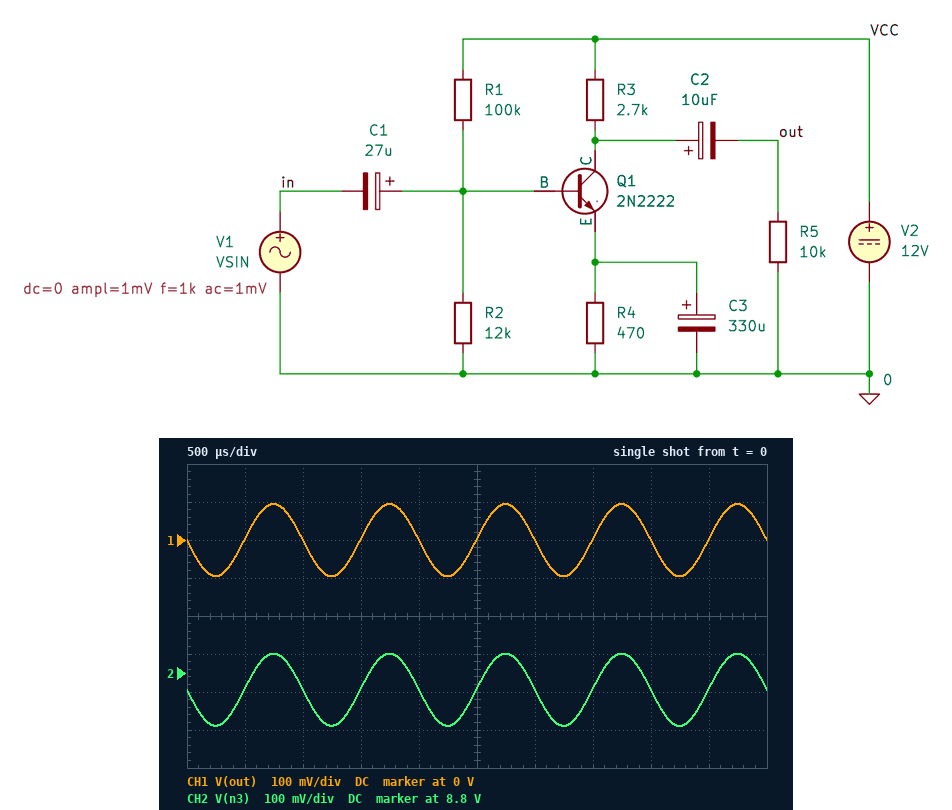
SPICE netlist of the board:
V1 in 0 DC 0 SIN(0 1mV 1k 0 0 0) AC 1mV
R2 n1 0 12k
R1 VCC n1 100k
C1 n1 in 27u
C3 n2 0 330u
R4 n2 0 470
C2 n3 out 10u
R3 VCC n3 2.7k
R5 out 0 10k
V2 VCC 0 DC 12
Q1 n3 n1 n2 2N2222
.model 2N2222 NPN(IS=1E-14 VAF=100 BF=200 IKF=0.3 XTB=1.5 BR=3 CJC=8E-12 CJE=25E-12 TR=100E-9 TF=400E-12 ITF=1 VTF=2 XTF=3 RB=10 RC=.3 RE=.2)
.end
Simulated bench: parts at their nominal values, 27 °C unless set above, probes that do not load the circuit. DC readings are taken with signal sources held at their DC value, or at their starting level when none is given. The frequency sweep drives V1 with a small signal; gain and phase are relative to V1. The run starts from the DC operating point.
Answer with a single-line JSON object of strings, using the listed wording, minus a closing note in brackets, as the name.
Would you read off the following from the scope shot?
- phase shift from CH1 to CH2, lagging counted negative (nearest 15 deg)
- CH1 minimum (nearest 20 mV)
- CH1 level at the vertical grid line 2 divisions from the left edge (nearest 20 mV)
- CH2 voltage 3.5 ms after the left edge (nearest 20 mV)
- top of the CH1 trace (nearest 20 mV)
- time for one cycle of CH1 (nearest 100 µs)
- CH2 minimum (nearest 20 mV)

{"phase shift from CH1 to CH2, lagging counted negative": "0 deg", "CH1 minimum": "-100 mV", "CH1 level at the vertical grid line 2 divisions from the left edge": "0 V", "CH2 voltage 3.5 ms after the left edge": "8.76 V", "top of the CH1 trace": "100 mV", "time for one cycle of CH1": "1.0 ms", "CH2 minimum": "8.66 V"}
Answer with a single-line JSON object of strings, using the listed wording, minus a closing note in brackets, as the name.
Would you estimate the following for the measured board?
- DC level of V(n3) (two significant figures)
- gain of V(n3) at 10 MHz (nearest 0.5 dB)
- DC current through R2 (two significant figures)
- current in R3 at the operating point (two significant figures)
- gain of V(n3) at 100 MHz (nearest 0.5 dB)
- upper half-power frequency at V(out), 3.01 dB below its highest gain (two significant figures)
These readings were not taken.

{"DC level of V(n3)": "8.8 V", "gain of V(n3) at 10 MHz": "38.0 dB", "DC current through R2": "100 µA", "current in R3 at the operating point": "1.2 mA", "gain of V(n3) at 100 MHz": "22.5 dB", "upper half-power frequency at V(out), 3.01 dB below its highest gain": "14 MHz"}
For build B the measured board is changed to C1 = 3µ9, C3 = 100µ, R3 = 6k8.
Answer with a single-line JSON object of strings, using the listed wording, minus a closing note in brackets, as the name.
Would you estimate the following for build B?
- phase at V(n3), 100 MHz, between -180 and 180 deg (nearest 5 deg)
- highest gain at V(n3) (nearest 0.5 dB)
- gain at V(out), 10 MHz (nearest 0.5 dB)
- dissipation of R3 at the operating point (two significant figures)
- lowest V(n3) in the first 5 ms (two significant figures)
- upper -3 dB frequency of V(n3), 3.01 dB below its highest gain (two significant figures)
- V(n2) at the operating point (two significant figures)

{"phase at V(n3), 100 MHz, between -180 and 180 deg": "75 deg", "highest gain at V(n3)": "45.0 dB", "gain at V(out), 10 MHz": "39.0 dB", "dissipation of R3 at the operating point": "9.7 mW", "lowest V(n3) in the first 5 ms": "3.7 V", "upper -3 dB frequency of V(n3), 3.01 dB below its highest gain": "5.8 MHz", "V(n2) at the operating point": "560 mV"}
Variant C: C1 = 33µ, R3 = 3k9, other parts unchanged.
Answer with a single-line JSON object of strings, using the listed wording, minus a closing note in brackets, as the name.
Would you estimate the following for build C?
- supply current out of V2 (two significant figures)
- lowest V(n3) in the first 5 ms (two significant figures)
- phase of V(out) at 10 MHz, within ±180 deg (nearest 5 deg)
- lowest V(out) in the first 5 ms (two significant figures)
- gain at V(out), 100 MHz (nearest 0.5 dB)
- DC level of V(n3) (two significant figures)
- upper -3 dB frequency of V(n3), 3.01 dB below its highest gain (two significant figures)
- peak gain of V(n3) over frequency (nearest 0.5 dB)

{"supply current out of V2": "1.3 mA", "lowest V(n3) in the first 5 ms": "7.2 V", "phase of V(out) at 10 MHz, within ±180 deg": "135 deg", "lowest V(out) in the first 5 ms": "-120 mV", "gain at V(out), 100 MHz": "22.0 dB", "DC level of V(n3)": "7.3 V", "upper -3 dB frequency of V(n3), 3.01 dB below its highest gain": "10 MHz", "peak gain of V(n3) over frequency": "42.0 dB"}
